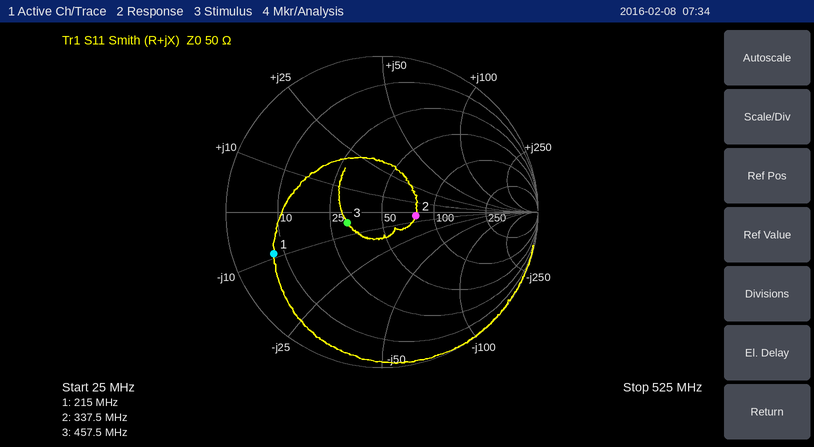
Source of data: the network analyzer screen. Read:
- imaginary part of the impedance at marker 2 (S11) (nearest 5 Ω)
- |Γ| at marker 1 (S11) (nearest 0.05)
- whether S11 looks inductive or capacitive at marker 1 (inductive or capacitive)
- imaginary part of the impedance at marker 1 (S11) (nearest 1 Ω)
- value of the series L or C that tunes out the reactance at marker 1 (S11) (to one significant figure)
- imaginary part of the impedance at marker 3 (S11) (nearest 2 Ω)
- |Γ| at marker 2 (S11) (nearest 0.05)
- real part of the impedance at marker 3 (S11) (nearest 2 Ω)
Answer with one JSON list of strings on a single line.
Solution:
["-5 Ω", "0.75", "capacitive", "-9 Ω", "7 nH", "-4 Ω", "0.20", "32 Ω"]
